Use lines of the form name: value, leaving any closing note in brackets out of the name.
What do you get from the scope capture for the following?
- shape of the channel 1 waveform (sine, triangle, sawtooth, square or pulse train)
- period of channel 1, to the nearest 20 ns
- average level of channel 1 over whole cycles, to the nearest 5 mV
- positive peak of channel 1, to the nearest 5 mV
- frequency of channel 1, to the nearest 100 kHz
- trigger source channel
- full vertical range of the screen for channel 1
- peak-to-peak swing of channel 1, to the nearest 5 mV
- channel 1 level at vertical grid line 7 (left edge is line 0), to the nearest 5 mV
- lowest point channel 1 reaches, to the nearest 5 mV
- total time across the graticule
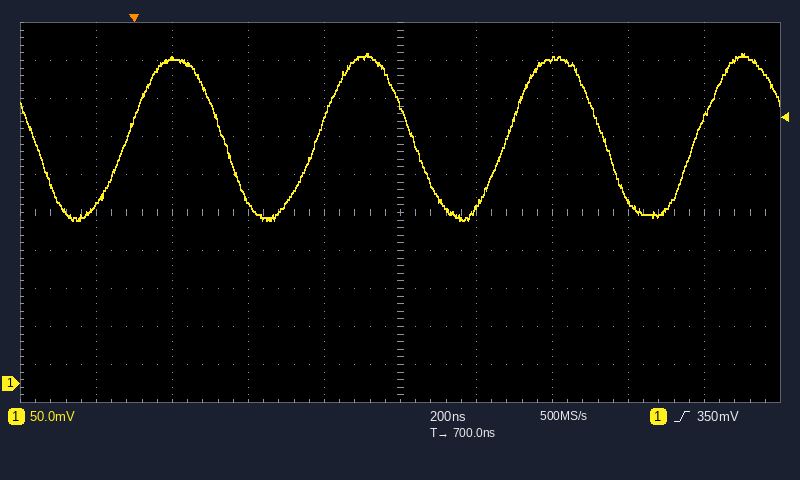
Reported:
shape of the channel 1 waveform: sine
period of channel 1, to the nearest 20 ns: 500 ns
average level of channel 1 over whole cycles, to the nearest 5 mV: 325 mV
positive peak of channel 1, to the nearest 5 mV: 435 mV
frequency of channel 1, to the nearest 100 kHz: 2.0 MHz
trigger source channel: channel 1
full vertical range of the screen for channel 1: 500 mV
peak-to-peak swing of channel 1, to the nearest 5 mV: 220 mV
channel 1 level at vertical grid line 7 (left edge is line 0), to the nearest 5 mV: 425 mV
lowest point channel 1 reaches, to the nearest 5 mV: 215 mV
total time across the graticule: 2 µs
